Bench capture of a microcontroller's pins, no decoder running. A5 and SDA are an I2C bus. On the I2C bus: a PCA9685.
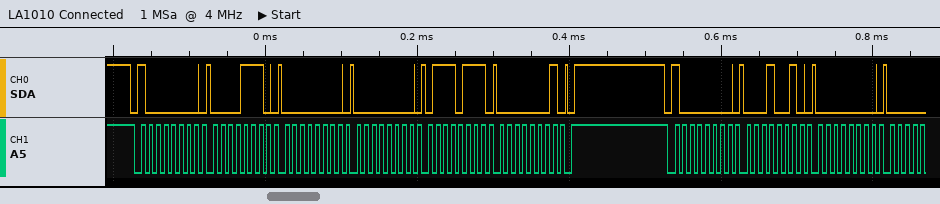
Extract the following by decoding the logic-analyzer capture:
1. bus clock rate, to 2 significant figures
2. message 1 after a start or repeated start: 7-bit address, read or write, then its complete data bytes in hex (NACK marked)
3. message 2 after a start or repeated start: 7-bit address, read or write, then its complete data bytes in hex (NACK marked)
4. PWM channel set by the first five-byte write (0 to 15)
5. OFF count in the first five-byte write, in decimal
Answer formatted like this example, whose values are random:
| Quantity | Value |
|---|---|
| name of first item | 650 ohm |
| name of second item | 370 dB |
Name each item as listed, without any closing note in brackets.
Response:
| Quantity | Value |
|---|---|
| bus clock rate, to 2 significant figures | 100 kHz |
| message 1 after a start or repeated start: 7-bit address, read or write, then its complete data bytes in hex | 0x40 write: 0E 00 00 77 01 |
| message 2 after a start or repeated start: 7-bit address, read or write, then its complete data bytes in hex | 0x40 write: 12 00 |
| PWM channel set by the first five-byte write | 2 |
| OFF count in the first five-byte write, in decimal | 375 |
